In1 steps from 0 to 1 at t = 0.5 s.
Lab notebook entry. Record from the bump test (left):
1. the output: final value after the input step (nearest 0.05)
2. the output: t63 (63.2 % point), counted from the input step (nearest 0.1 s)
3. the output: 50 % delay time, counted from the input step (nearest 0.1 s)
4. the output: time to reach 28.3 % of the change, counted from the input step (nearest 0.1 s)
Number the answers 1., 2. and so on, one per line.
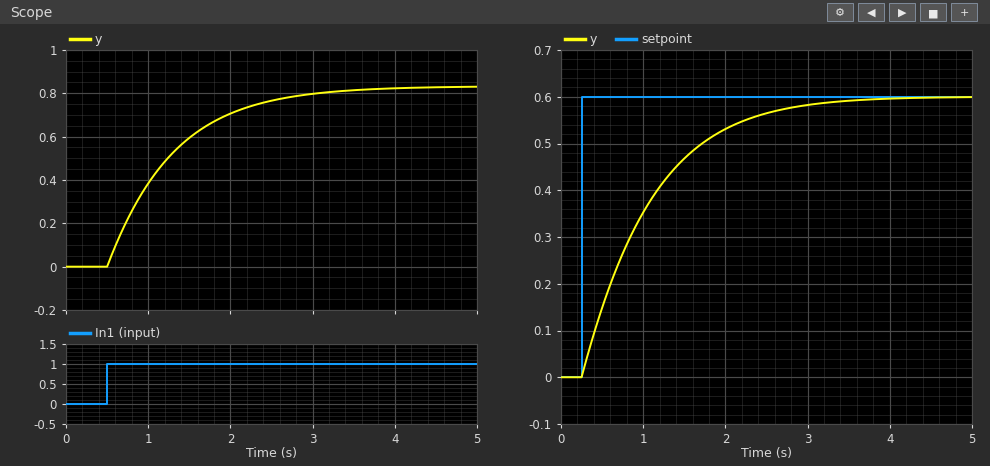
1. 0.85
2. 0.8 s
3. 0.6 s
4. 0.3 s
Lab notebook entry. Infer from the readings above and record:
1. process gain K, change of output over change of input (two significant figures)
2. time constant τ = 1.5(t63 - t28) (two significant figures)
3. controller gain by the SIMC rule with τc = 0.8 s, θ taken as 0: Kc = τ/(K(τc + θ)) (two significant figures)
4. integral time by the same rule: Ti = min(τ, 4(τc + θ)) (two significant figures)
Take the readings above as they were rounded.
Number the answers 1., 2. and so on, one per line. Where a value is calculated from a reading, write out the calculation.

1. (0.85 - 0) / 1 = 0.85
2. 1.5 × (0.8 - 0.3) = 0.75 s
3. 0.75 / (0.85 × (0.8 + 0)) = 1.1
4. min(0.75, 4 × (0.8 + 0)) = 0.75 s
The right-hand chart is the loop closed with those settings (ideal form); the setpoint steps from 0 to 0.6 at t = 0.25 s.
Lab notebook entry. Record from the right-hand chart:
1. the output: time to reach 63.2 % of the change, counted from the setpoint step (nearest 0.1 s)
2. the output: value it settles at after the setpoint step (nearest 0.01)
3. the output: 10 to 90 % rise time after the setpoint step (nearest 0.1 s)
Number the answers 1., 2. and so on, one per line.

1. 0.8 s
2. 0.60
3. 1.8 s
